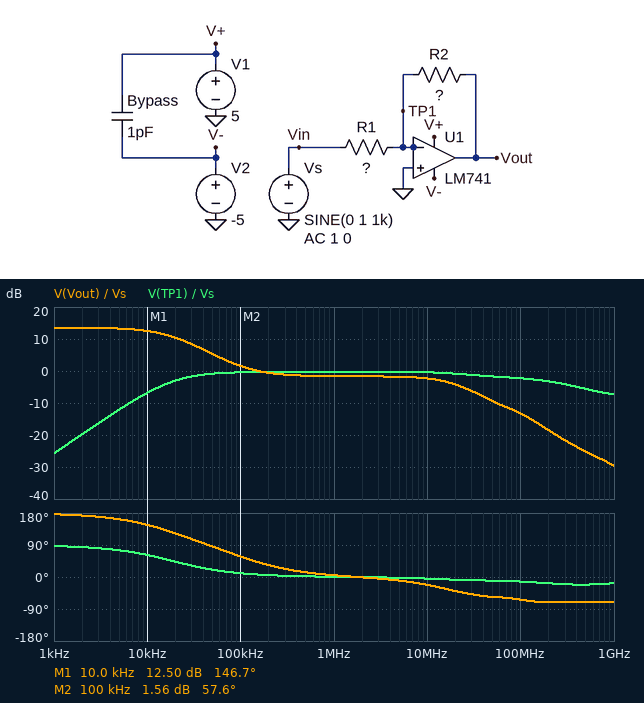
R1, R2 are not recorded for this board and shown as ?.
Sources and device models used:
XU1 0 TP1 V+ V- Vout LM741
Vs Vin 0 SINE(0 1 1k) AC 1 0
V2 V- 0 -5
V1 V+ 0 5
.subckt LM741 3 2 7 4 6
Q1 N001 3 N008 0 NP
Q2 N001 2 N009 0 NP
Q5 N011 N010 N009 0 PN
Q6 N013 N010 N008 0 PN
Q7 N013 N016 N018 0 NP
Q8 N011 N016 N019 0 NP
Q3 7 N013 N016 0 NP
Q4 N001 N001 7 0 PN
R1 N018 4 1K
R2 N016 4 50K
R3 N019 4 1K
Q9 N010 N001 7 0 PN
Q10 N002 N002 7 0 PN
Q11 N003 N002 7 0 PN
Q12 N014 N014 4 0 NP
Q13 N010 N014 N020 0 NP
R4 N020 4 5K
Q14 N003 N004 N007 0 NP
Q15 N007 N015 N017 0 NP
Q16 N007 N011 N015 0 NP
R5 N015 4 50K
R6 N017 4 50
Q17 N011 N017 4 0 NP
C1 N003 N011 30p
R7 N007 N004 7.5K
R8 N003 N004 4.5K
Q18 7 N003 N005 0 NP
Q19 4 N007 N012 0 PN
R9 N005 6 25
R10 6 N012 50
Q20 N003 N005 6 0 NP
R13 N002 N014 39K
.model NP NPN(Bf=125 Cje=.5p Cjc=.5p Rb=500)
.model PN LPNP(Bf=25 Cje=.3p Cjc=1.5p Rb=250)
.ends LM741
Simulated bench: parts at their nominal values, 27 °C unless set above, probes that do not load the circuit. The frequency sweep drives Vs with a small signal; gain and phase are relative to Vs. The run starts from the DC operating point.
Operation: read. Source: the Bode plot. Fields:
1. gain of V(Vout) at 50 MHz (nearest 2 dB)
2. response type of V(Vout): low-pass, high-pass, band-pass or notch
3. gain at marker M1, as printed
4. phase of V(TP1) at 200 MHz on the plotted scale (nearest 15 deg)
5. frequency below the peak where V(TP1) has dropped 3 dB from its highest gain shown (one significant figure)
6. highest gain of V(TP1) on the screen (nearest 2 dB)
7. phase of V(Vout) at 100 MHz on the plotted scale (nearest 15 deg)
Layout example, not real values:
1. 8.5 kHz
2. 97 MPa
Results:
1. -10 dB
2. low-pass
3. 12.50 dB
4. -15 deg
5. 20 kHz
6. 0 dB
7. -60 deg
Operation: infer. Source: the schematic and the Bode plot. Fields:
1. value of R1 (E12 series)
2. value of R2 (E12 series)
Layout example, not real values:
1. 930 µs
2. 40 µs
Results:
1. 820 Ω
2. 3.9 kΩ
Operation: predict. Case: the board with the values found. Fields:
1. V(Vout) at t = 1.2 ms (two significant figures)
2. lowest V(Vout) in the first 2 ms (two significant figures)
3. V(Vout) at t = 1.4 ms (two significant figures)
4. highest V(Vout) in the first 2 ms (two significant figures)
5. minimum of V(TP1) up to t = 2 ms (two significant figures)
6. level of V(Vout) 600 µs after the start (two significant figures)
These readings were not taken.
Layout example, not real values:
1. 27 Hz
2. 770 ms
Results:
1. -3.4 V
2. -3.4 V
3. -2.8 V
4. 4.2 V
5. -100 mV
6. 2.8 V
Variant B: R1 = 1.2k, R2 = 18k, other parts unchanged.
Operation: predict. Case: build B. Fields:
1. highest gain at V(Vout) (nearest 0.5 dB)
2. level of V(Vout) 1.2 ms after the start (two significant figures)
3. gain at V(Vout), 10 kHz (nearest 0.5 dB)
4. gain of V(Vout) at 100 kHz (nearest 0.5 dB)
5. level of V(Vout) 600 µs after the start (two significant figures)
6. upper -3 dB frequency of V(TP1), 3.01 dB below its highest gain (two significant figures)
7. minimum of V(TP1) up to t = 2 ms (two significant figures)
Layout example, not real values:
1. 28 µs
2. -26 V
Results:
1. 23.5 dB
2. -3.5 V
3. 22.5 dB
4. 9.0 dB
5. 4.2 V
6. 190 MHz
7. -670 mV
